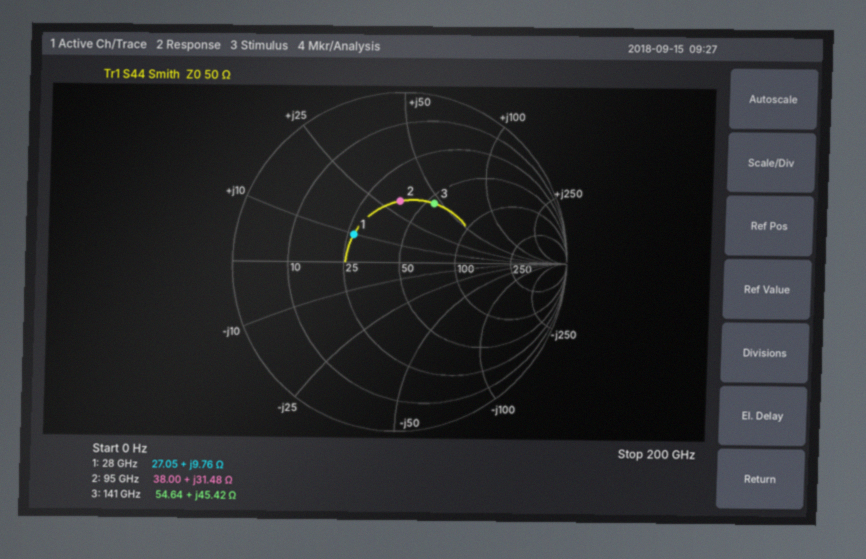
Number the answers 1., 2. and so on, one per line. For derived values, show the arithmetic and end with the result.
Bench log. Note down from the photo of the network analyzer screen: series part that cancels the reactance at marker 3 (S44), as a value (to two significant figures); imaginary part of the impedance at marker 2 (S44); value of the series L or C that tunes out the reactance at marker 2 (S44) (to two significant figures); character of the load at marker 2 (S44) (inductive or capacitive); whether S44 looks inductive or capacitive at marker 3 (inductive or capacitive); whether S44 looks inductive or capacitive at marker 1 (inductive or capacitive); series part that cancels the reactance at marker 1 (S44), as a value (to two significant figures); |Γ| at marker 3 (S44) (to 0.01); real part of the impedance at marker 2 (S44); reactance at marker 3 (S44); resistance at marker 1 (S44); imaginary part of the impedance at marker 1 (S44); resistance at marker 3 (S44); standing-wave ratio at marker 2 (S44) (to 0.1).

1. C = 1/(2π × 141 GHz × 45.42 Ω) ≈ 25 fF
2. +31.48 Ω
3. C = 1/(2π × 95 GHz × 31.48 Ω) ≈ 53 fF
4. inductive
5. inductive
6. inductive
7. C = 1/(2π × 28 GHz × 9.76 Ω) ≈ 582 fF, so 580 fF to two significant figures
8. 0.40
9. 38.00 Ω
10. +45.42 Ω
11. 27.05 Ω
12. +9.76 Ω
13. 54.64 Ω
14. 2.1
